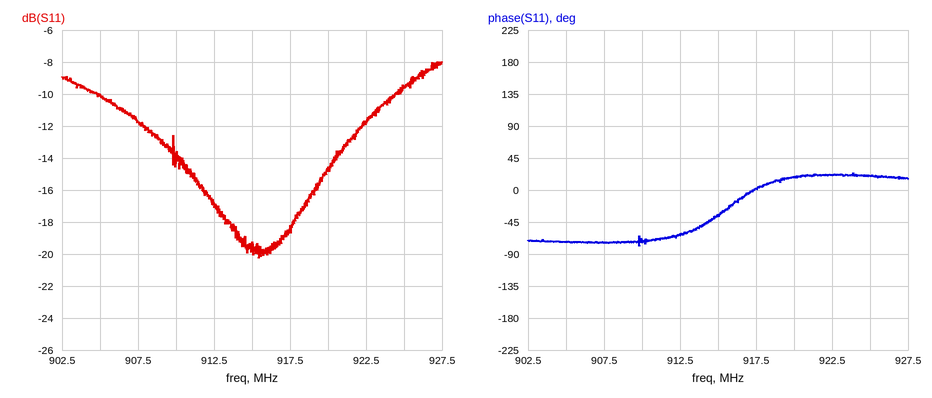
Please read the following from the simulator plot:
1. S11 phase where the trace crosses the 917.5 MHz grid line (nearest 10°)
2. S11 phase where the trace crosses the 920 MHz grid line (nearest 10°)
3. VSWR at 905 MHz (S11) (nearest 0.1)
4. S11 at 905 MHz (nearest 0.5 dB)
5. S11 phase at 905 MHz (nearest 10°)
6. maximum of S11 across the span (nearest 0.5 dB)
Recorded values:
0°
20°
1.9
-10.0 dB
-70°
-8.0 dB
